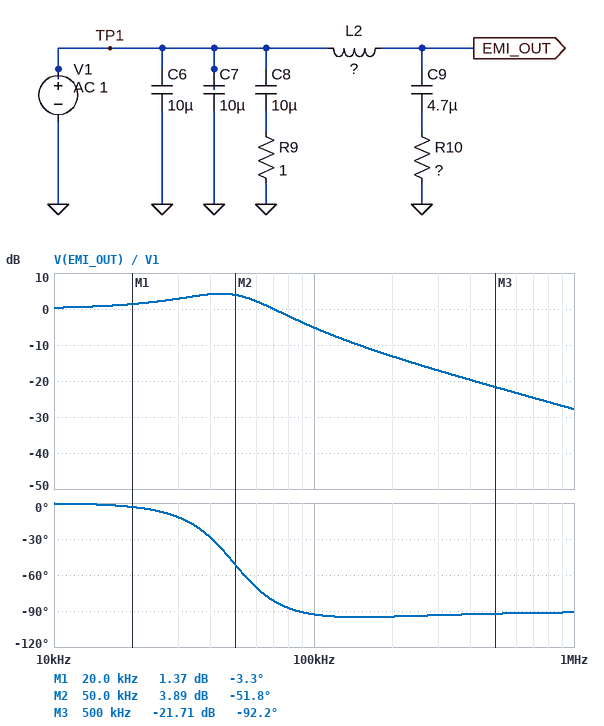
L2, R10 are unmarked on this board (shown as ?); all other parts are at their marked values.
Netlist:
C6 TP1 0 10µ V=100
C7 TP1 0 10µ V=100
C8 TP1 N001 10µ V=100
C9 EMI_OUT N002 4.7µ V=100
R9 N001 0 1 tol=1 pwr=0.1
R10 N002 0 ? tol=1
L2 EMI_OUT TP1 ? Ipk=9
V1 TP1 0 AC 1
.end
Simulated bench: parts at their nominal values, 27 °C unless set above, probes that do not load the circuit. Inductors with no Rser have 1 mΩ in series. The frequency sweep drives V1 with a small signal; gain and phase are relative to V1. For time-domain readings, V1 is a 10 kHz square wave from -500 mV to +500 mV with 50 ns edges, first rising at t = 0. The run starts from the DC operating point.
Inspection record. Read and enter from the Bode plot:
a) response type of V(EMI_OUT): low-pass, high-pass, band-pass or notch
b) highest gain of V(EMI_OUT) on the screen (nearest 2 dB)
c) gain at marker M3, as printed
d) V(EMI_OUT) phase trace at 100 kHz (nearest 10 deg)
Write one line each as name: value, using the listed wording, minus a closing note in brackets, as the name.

response type of V(EMI_OUT): low-pass, high-pass, band-pass or notch: low-pass
highest gain of V(EMI_OUT) on the screen: 4 dB
gain at marker M3, as printed: -21.71 dB
V(EMI_OUT) phase trace at 100 kHz: -90 deg
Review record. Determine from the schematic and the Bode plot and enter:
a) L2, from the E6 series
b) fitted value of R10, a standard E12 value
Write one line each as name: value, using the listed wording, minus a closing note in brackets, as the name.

L2, from the E6 series: 2.2 µH
fitted value of R10, a standard E12 value: 0.56 Ω
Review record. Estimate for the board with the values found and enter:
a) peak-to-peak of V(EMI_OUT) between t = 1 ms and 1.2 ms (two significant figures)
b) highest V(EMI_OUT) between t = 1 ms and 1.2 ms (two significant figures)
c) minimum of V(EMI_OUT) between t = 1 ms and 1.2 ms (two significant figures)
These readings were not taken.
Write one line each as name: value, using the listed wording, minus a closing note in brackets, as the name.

peak-to-peak of V(EMI_OUT) between t = 1 ms and 1.2 ms: 1.7 V
highest V(EMI_OUT) between t = 1 ms and 1.2 ms: 860 mV
minimum of V(EMI_OUT) between t = 1 ms and 1.2 ms: -860 mV
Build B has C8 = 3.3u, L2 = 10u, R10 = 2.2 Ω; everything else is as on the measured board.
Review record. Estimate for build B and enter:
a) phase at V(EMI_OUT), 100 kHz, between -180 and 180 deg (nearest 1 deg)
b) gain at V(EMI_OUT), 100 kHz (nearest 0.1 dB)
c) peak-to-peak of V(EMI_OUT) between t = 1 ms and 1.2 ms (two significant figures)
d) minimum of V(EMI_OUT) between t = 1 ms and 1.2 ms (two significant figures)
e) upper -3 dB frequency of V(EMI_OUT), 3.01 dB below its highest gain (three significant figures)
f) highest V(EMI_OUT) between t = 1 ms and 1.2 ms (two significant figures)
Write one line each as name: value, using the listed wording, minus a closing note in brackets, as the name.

phase at V(EMI_OUT), 100 kHz, between -180 and 180 deg: -78 deg
gain at V(EMI_OUT), 100 kHz: -9.1 dB
peak-to-peak of V(EMI_OUT) between t = 1 ms and 1.2 ms: 1.4 V
minimum of V(EMI_OUT) between t = 1 ms and 1.2 ms: -690 mV
upper -3 dB frequency of V(EMI_OUT), 3.01 dB below its highest gain: 38.6 kHz
highest V(EMI_OUT) between t = 1 ms and 1.2 ms: 690 mV
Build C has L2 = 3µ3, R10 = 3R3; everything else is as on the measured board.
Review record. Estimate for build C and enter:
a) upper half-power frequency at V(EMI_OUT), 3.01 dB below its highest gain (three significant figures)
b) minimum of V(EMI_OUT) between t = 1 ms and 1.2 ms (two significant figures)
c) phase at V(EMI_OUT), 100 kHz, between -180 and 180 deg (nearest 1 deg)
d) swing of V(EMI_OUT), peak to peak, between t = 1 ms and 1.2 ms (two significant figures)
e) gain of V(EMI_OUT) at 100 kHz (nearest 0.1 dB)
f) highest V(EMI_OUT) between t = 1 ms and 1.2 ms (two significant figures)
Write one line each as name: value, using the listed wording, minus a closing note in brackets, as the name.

upper half-power frequency at V(EMI_OUT), 3.01 dB below its highest gain: 155 kHz
minimum of V(EMI_OUT) between t = 1 ms and 1.2 ms: -550 mV
phase at V(EMI_OUT), 100 kHz, between -180 and 180 deg: -34 deg
swing of V(EMI_OUT), peak to peak, between t = 1 ms and 1.2 ms: 1.1 V
gain of V(EMI_OUT) at 100 kHz: -1.0 dB
highest V(EMI_OUT) between t = 1 ms and 1.2 ms: 550 mV
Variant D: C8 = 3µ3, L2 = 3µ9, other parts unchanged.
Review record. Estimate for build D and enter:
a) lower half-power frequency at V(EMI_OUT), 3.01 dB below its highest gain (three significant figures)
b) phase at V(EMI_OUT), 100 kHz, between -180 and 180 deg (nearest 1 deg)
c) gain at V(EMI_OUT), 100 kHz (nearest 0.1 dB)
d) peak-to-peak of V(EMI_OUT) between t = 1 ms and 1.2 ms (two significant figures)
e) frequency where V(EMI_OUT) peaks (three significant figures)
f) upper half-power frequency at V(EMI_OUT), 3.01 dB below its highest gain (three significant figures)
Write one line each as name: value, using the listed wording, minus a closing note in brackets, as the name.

lower half-power frequency at V(EMI_OUT), 3.01 dB below its highest gain: 21.0 kHz
phase at V(EMI_OUT), 100 kHz, between -180 and 180 deg: -106 deg
gain at V(EMI_OUT), 100 kHz: -10.5 dB
peak-to-peak of V(EMI_OUT) between t = 1 ms and 1.2 ms: 1.9 V
frequency where V(EMI_OUT) peaks: 34.5 kHz
upper half-power frequency at V(EMI_OUT), 3.01 dB below its highest gain: 45.5 kHz
